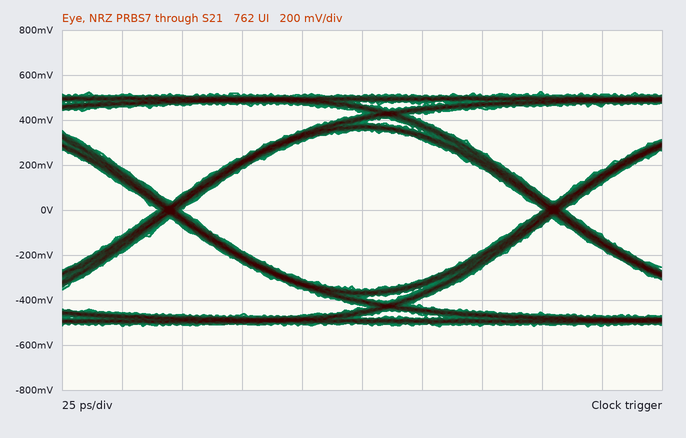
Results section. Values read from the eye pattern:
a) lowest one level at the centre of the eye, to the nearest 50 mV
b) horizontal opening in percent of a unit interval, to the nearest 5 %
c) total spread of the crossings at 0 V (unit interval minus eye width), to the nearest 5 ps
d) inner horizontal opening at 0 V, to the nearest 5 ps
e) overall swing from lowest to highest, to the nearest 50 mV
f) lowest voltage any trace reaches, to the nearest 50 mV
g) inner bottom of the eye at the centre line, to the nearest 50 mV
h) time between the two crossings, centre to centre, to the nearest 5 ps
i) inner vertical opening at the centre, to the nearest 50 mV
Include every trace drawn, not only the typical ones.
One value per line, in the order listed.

350 mV
95 %
10 ps
150 ps
1.05 V
-500 mV
-350 mV
160 ps
700 mV
